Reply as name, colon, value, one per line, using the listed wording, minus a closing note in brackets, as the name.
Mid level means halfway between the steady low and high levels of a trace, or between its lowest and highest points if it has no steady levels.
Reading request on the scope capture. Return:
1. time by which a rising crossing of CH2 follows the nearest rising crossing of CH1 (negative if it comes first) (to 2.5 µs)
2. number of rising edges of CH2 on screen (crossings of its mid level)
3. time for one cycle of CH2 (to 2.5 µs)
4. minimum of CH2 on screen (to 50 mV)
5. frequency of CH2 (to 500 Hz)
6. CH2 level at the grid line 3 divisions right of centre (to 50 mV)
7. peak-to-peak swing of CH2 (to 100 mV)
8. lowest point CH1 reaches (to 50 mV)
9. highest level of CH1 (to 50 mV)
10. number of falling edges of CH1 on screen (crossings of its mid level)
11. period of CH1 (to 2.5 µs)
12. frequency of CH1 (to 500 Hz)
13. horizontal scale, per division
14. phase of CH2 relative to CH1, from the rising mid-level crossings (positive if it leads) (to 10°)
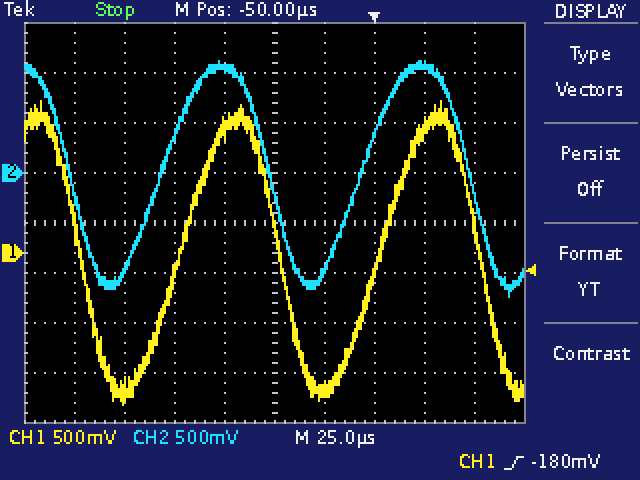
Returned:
time by which a rising crossing of CH2 follows the nearest rising crossing of CH1 (negative if it comes first): -10.0 µs
number of rising edges of CH2 on screen: 2
time for one cycle of CH2: 100.0 µs
minimum of CH2 on screen: -1.25 V
frequency of CH2: 10.0 kHz
CH2 level at the grid line 3 divisions right of centre: 1.10 V
peak-to-peak swing of CH2: 2.40 V
lowest point CH1 reaches: -1.50 V
highest level of CH1: 1.50 V
number of falling edges of CH1 on screen: 3
period of CH1: 100.0 µs
frequency of CH1: 10.0 kHz
horizontal scale, per division: 25 µs
phase of CH2 relative to CH1, from the rising mid-level crossings (positive if it leads): +40°
